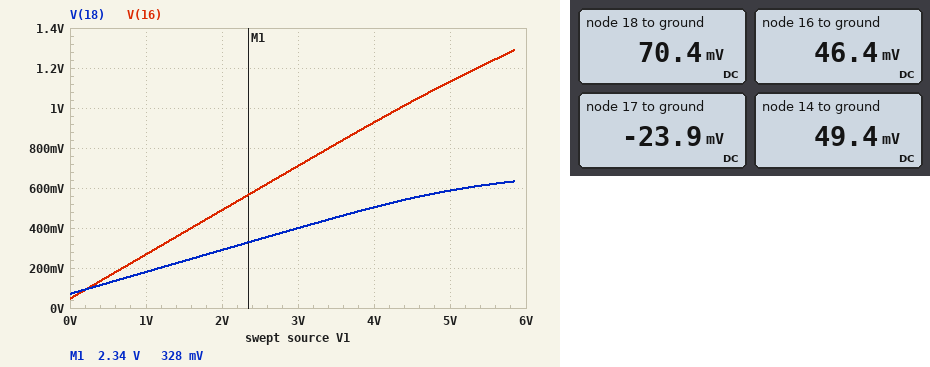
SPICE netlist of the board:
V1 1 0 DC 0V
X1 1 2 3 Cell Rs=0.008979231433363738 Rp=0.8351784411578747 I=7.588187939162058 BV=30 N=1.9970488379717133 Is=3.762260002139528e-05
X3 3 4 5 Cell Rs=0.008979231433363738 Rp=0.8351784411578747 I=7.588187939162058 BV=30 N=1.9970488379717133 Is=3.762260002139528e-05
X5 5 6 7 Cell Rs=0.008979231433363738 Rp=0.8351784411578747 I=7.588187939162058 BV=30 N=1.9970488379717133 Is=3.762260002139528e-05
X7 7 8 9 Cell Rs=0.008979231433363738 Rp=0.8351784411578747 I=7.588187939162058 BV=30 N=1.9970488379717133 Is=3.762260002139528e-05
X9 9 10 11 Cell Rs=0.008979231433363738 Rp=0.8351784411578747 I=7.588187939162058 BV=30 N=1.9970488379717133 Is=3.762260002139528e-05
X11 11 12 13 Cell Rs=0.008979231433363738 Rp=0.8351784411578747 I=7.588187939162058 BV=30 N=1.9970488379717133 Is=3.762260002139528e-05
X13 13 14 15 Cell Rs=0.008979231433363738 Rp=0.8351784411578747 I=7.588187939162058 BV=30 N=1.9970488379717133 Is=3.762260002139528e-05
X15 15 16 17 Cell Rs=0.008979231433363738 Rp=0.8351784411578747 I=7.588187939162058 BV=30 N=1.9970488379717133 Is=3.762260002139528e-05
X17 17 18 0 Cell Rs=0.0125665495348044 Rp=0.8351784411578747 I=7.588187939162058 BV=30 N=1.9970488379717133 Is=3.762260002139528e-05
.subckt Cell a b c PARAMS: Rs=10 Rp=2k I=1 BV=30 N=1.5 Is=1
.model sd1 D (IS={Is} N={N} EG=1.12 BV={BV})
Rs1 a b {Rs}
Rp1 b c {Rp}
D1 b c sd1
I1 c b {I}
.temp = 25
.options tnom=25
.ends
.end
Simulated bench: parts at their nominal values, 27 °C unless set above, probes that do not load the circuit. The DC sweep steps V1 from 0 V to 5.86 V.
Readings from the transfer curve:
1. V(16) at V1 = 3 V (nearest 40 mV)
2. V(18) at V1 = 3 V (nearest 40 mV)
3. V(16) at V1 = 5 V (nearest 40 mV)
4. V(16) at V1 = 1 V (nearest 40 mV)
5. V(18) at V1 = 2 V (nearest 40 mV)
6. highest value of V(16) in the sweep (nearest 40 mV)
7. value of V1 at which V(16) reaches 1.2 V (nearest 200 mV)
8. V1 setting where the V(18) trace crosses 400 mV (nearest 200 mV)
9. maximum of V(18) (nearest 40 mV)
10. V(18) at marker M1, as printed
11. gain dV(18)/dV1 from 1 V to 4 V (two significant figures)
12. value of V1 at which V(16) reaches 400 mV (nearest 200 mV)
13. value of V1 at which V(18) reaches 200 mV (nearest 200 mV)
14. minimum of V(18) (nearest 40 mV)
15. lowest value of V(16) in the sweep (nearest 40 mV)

720 mV
400 mV
1.12 V
280 mV
280 mV
1.28 V
5.4 V
3.0 V
640 mV
328 mV
0.11 V/V
1.6 V
1.2 V
80 mV
40 mV
